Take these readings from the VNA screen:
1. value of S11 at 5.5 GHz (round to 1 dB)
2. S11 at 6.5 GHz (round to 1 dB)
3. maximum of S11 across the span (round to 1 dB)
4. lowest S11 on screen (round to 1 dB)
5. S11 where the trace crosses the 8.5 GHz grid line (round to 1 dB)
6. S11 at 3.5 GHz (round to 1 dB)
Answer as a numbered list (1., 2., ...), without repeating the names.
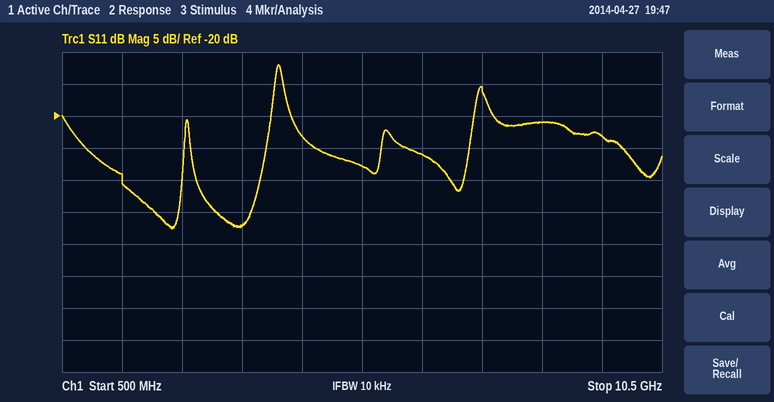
1. -28 dB
2. -26 dB
3. -12 dB
4. -38 dB
5. -21 dB
6. -37 dB
